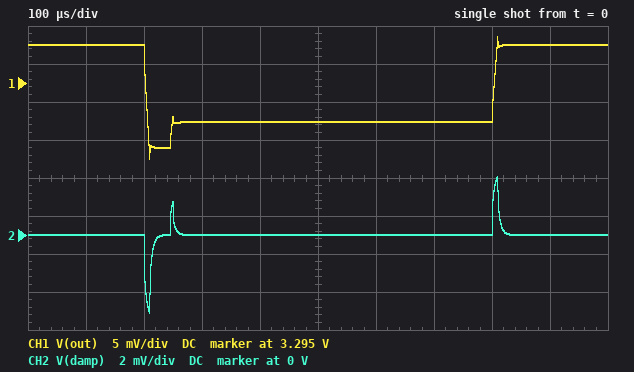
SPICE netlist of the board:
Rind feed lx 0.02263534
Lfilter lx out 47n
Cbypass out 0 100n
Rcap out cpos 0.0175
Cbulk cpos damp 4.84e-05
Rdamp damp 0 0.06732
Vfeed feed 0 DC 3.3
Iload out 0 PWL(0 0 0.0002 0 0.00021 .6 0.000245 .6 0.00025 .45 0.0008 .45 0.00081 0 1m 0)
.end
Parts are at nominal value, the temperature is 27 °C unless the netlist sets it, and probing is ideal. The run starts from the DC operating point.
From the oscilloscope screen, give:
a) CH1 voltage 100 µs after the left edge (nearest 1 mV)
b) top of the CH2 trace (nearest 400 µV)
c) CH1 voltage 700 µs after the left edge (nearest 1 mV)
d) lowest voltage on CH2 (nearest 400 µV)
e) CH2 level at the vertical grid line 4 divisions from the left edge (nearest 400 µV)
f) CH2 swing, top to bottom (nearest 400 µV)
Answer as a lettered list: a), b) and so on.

a) 3.300 V
b) 3.2 mV
c) 3.290 V
d) -4.0 mV
e) 0 V
f) 7.2 mV
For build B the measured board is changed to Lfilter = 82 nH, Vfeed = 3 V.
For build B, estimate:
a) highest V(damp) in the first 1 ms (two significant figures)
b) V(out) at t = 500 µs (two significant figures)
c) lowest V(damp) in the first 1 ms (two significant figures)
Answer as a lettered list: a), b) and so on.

a) 3.3 mV
b) 3.0 V
c) -4.3 mV
